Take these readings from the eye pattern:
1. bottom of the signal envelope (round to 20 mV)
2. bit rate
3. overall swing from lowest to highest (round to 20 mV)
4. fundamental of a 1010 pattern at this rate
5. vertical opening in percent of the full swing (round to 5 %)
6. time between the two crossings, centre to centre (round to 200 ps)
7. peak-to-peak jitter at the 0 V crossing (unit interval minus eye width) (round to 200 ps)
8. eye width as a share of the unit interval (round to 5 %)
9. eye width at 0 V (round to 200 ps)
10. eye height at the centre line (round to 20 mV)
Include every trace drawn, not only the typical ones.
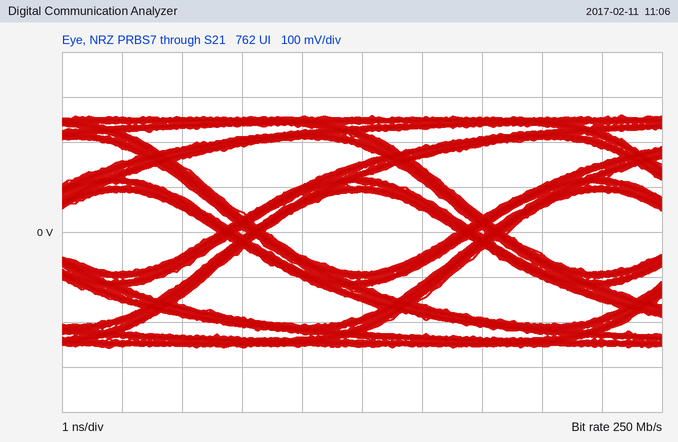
-260 mV
250 Mb/s
520 mV
125 MHz
35 %
4.0 ns
800 ps
80 %
3.2 ns
180 mV
